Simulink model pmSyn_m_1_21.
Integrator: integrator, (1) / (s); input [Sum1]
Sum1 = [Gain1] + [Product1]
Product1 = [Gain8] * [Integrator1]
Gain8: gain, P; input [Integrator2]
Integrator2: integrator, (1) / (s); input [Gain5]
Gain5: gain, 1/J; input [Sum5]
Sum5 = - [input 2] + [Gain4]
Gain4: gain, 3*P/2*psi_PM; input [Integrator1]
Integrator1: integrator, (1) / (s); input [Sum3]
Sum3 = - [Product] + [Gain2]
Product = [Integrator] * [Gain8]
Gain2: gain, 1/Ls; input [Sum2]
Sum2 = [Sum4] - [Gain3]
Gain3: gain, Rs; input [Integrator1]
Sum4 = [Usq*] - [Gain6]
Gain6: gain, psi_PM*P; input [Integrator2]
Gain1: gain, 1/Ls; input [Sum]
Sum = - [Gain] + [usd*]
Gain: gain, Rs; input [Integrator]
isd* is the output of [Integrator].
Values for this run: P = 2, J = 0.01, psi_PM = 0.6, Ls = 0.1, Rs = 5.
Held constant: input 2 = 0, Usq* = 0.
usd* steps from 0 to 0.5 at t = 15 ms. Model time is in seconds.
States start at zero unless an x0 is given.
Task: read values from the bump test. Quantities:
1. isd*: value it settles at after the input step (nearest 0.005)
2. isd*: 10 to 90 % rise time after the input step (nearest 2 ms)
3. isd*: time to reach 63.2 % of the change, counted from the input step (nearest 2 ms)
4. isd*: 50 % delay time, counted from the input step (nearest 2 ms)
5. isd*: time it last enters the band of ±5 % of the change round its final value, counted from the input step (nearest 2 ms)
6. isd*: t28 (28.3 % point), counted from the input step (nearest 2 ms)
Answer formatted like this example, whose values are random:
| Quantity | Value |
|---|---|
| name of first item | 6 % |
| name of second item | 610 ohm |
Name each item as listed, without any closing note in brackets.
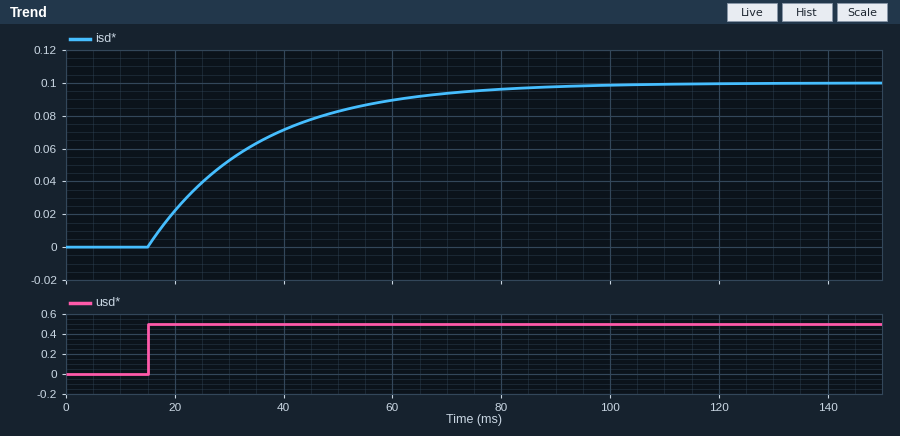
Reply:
| Quantity | Value |
|---|---|
| isd*: value it settles at after the input step | 0.100 |
| isd*: 10 to 90 % rise time after the input step | 44 ms |
| isd*: time to reach 63.2 % of the change, counted from the input step | 20 ms |
| isd*: 50 % delay time, counted from the input step | 14 ms |
| isd*: time it last enters the band of ±5 % of the change round its final value, counted from the input step | 60 ms |
| isd*: t28 (28.3 % point), counted from the input step | 6 ms |
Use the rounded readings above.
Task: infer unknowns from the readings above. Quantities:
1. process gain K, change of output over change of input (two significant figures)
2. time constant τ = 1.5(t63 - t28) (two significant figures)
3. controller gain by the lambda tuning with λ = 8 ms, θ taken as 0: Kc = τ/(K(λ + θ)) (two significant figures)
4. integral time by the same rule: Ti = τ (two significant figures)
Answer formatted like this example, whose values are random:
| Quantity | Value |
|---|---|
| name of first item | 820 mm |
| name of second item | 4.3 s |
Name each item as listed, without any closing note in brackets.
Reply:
| Quantity | Value |
|---|---|
| process gain K, change of output over change of input | 0.20 |
| time constant τ = 1.5(t63 - t28) | 21 ms |
| controller gain by the lambda tuning with λ = 8 ms, θ taken as 0: Kc = τ/(K(λ + θ)) | 13 |
| integral time by the same rule: Ti = τ | 21 ms |
